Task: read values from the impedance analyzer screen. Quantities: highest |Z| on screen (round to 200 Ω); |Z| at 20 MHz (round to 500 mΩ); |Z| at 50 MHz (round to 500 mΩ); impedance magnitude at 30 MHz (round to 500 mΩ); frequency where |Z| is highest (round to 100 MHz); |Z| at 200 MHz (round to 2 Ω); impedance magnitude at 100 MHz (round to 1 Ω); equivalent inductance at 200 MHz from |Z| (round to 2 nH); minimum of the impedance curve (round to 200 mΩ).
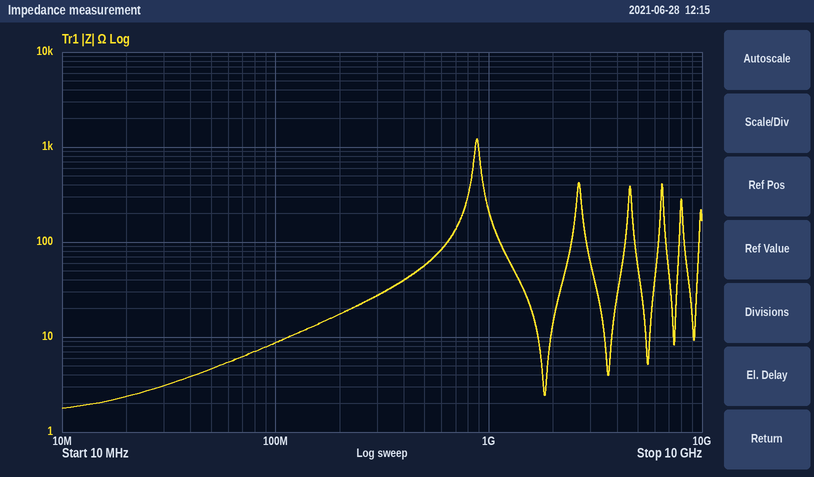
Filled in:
1.2 kΩ
2.5 Ω
4.5 Ω
3.0 Ω
900 MHz
18 Ω
9 Ω
14 nH
1.8 Ω
